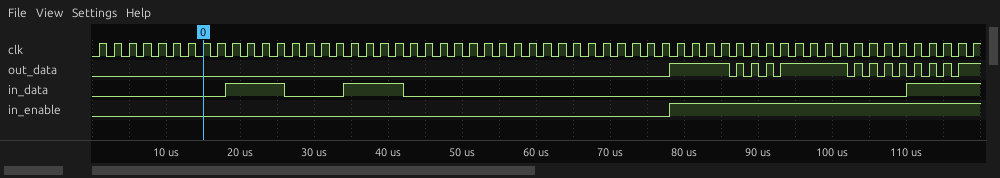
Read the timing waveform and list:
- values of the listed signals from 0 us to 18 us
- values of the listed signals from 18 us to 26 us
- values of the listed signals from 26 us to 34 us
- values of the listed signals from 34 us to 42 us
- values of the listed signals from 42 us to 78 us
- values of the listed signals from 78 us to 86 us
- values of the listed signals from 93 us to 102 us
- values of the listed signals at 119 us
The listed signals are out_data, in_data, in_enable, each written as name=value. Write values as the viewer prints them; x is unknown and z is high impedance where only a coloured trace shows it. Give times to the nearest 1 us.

out_data=0, in_data=0, in_enable=0
out_data=0, in_data=1, in_enable=0
out_data=0, in_data=0, in_enable=0
out_data=0, in_data=1, in_enable=0
out_data=0, in_data=0, in_enable=0
out_data=1, in_data=0, in_enable=1
out_data=1, in_data=0, in_enable=1
out_data=1, in_data=1, in_enable=1
